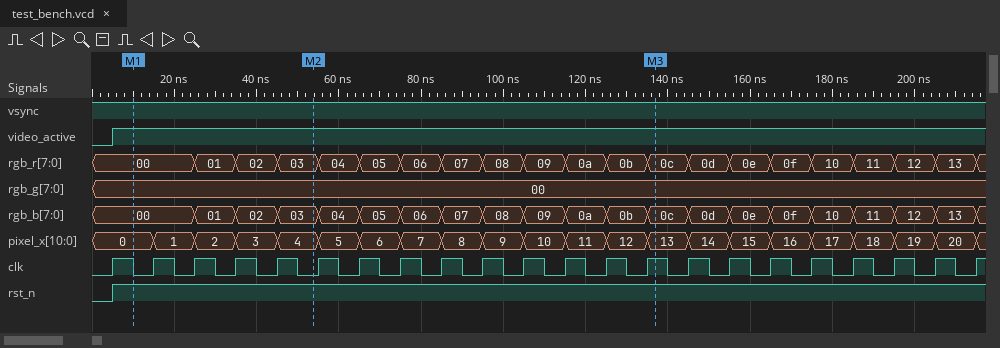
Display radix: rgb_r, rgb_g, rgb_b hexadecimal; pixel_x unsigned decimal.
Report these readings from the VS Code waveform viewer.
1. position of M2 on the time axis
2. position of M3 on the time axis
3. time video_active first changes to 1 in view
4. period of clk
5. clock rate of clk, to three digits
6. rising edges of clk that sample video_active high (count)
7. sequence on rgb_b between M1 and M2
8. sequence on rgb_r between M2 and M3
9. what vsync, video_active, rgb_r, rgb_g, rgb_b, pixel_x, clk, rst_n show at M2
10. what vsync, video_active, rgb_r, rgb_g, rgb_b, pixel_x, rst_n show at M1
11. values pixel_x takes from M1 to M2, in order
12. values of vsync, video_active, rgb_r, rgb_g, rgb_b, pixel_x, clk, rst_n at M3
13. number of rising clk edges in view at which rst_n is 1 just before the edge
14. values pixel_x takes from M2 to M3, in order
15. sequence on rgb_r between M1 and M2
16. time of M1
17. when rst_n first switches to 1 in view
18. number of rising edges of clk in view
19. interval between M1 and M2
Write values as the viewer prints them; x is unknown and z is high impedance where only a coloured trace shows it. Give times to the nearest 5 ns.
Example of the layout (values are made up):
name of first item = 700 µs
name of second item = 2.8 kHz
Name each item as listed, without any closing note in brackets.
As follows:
position of M2 on the time axis = 55 ns
position of M3 on the time axis = 135 ns
time video_active first changes to 1 in view = 5 ns
period of clk = 10 ns
clock rate of clk, to three digits = 100 MHz
rising edges of clk that sample video_active high = 21
sequence on rgb_b between M1 and M2 = 00, 01, 02, 03
sequence on rgb_r between M2 and M3 = 03, 04, 05, 06, 07, 08, 09, 0a, 0b, 0c
what vsync, video_active, rgb_r, rgb_g, rgb_b, pixel_x, clk, rst_n show at M2 = vsync=1, video_active=1, rgb_r=03, rgb_g=00, rgb_b=03, pixel_x=4, clk=0, rst_n=1
what vsync, video_active, rgb_r, rgb_g, rgb_b, pixel_x, rst_n show at M1 = vsync=1, video_active=1, rgb_r=00, rgb_g=00, rgb_b=00, pixel_x=0, rst_n=1
values pixel_x takes from M1 to M2, in order = 0, 1, 2, 3, 4
values of vsync, video_active, rgb_r, rgb_g, rgb_b, pixel_x, clk, rst_n at M3 = vsync=1, video_active=1, rgb_r=0c, rgb_g=00, rgb_b=0c, pixel_x=13, clk=1, rst_n=1
number of rising clk edges in view at which rst_n is 1 just before the edge = 21
values pixel_x takes from M2 to M3, in order = 4, 5, 6, 7, 8, 9, 10, 11, 12, 13
sequence on rgb_r between M1 and M2 = 00, 01, 02, 03
time of M1 = 10 ns
when rst_n first switches to 1 in view = 5 ns
number of rising edges of clk in view = 22
interval between M1 and M2 = 45 ns
